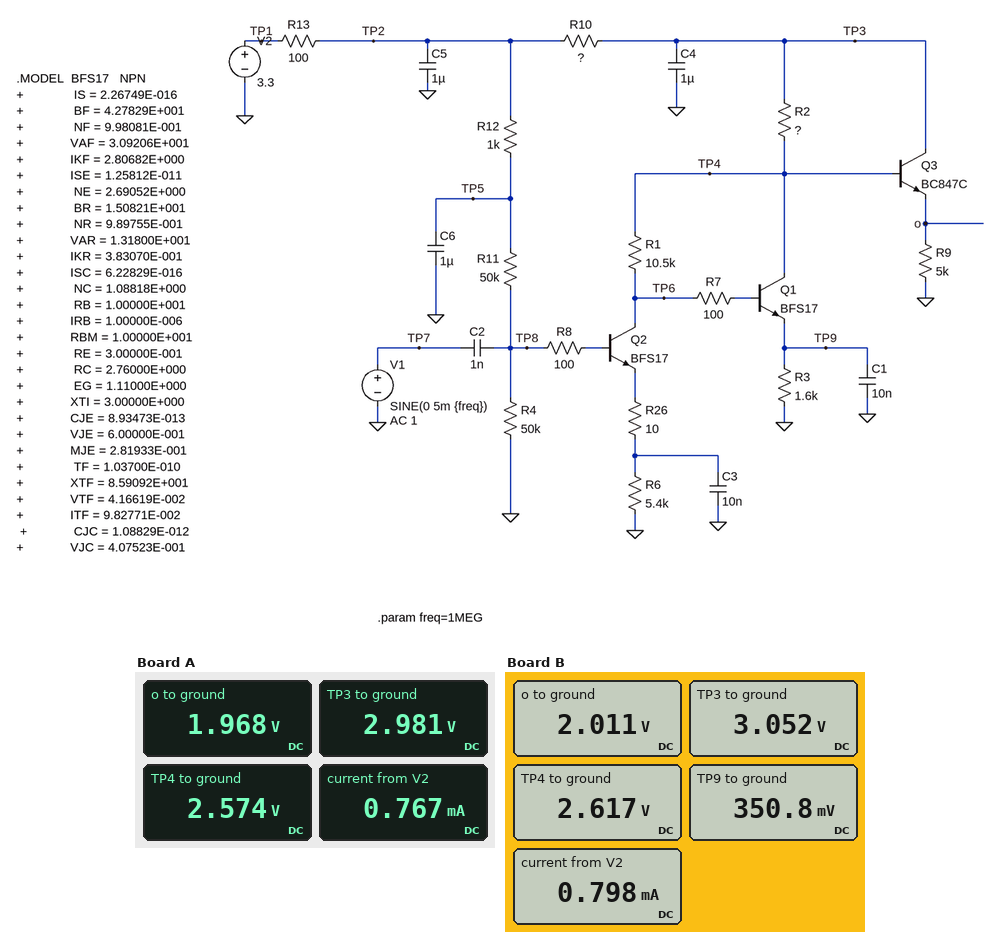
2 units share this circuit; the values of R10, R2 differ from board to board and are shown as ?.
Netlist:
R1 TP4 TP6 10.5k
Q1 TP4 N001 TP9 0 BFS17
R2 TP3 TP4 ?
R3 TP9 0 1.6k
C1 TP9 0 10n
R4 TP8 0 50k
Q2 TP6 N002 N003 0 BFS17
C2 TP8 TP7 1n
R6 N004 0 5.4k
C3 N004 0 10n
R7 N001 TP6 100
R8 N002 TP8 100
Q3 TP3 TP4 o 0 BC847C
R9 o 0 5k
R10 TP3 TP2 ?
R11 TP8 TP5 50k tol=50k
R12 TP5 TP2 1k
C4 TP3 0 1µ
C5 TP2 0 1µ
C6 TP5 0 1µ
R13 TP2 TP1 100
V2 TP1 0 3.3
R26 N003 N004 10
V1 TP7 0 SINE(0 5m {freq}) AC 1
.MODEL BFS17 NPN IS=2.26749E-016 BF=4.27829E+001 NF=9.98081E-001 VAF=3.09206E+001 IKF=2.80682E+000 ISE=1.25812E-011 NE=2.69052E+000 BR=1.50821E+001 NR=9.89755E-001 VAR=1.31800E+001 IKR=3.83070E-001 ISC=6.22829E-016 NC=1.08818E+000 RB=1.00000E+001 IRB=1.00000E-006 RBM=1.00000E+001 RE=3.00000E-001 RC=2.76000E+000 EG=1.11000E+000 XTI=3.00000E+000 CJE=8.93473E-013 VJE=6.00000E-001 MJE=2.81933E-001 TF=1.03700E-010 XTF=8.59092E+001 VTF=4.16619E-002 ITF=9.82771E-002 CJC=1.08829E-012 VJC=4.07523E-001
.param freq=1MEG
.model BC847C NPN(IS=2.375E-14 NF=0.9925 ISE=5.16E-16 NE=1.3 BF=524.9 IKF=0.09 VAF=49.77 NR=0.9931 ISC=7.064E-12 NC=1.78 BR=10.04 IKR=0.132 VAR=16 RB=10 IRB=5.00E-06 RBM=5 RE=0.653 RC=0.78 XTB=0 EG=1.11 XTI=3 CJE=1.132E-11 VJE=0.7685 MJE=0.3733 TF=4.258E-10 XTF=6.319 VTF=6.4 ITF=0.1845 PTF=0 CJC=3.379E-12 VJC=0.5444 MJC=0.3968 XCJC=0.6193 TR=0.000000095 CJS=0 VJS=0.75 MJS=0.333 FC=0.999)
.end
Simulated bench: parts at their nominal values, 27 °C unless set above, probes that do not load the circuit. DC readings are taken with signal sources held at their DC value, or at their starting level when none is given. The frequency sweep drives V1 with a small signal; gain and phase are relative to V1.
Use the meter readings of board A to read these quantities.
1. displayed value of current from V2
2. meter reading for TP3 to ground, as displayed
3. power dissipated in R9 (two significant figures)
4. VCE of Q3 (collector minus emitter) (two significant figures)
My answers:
0.767 mA
2.981 V
770 µW
1.0 V
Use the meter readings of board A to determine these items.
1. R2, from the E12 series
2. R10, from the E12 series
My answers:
1.2 kΩ
330 Ω
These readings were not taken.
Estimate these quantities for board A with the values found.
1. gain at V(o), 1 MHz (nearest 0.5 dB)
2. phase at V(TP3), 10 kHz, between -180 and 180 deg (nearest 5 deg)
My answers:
31.5 dB
35 deg
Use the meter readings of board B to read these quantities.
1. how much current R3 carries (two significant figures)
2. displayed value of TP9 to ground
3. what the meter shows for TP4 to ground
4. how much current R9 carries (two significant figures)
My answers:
220 µA
350.8 mV
2.617 V
400 µA
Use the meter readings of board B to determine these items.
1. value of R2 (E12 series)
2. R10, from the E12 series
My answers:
1.2 kΩ
220 Ω
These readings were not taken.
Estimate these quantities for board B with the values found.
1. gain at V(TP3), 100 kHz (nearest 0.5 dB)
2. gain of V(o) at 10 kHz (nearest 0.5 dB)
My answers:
-31.5 dB
5.5 dB
